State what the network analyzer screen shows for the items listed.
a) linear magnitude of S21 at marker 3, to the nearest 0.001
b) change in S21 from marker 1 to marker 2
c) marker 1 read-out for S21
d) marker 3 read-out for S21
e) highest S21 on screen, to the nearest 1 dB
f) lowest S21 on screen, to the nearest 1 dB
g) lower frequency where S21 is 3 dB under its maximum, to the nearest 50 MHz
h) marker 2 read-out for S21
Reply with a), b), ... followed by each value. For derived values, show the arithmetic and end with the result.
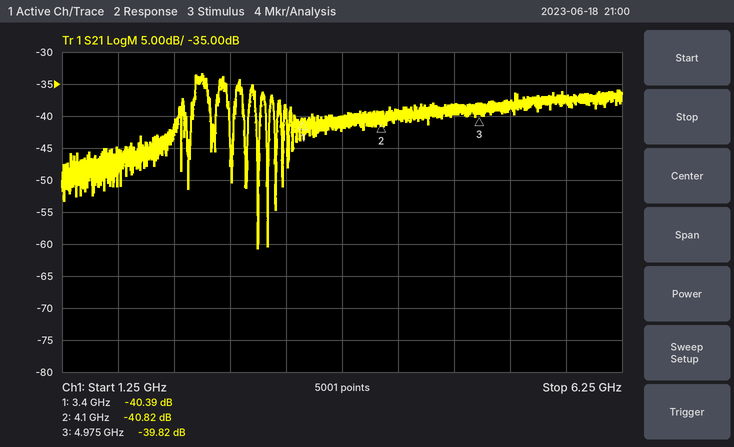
a) 10^(-39.82/20) ≈ 0.010
b) -40.82 − (-40.39) = -0.43 dB
c) -40.39 dB
d) -39.82 dB
e) -33 dB
f) -61 dB
g) 2.45 GHz
h) -40.82 dB
